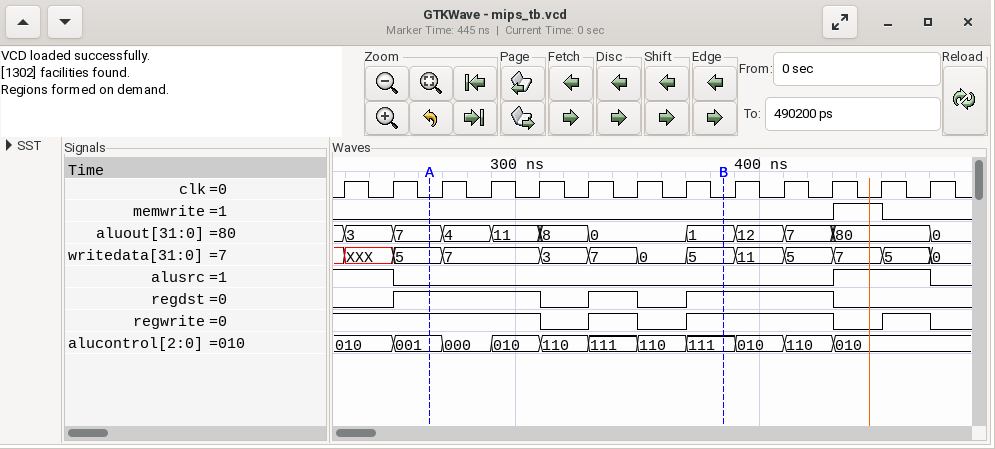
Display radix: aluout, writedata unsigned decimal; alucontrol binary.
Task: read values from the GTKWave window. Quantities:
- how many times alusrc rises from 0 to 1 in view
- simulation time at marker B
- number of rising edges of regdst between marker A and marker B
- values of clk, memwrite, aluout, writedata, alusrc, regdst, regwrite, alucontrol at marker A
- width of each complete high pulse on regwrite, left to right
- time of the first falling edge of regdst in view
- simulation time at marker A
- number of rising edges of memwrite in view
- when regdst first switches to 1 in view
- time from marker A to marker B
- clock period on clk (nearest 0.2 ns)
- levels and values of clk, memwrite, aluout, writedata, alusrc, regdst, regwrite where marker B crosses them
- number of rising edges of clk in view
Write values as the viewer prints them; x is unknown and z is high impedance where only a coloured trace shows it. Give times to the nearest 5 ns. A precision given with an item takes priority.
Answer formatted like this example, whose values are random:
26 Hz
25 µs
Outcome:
1
385 ns
2
clk=0, memwrite=0, aluout=7, writedata=5, alusrc=0, regdst=1, regwrite=1, alucontrol=001
20 ns, 60 ns, 20 ns
310 ns
265 ns
1
250 ns
120 ns
20 ns
clk=0, memwrite=0, aluout=1, writedata=5, alusrc=0, regdst=1, regwrite=1
13
